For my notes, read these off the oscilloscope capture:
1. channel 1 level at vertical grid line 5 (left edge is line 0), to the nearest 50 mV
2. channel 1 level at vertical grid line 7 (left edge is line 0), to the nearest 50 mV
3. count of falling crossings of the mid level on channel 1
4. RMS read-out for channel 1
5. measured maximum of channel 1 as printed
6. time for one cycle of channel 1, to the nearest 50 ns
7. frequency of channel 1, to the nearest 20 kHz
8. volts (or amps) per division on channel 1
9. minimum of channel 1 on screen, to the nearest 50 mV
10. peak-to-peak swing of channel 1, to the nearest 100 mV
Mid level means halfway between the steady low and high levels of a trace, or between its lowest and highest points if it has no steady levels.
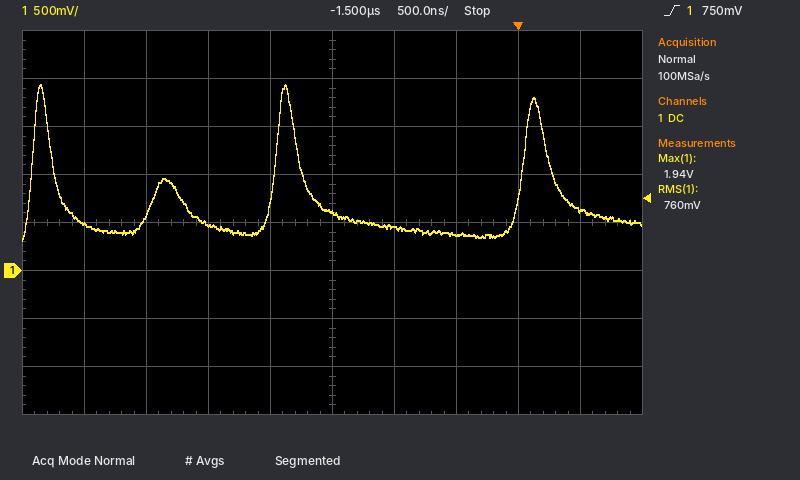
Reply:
600 mV
350 mV
3
760 mV
1.94 V
2.00 µs
500 kHz
500 mV
300 mV
1.60 V
